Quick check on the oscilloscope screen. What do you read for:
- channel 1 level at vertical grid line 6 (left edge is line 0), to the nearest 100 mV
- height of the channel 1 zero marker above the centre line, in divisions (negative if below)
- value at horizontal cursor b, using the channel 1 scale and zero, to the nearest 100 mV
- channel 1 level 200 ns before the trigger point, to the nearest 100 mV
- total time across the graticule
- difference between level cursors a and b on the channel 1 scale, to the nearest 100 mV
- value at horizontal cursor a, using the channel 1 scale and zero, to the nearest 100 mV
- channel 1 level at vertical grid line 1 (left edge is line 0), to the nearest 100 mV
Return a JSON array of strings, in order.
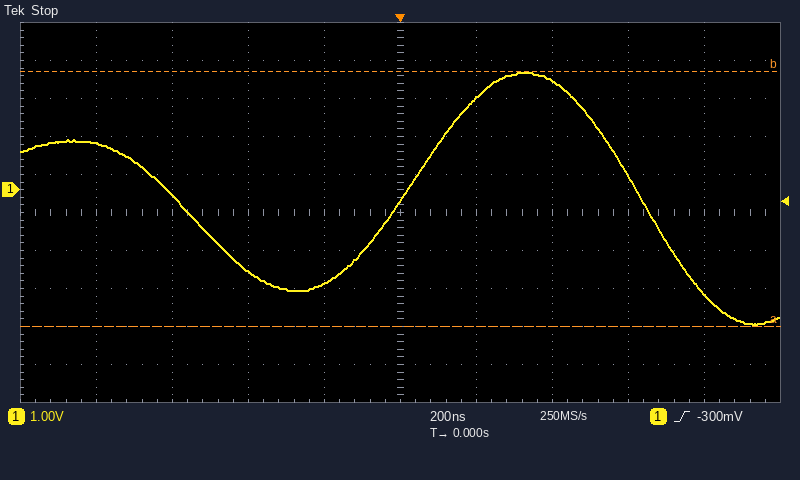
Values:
["2.4 V", "+0.6 div", "3.1 V", "-2.5 V", "2 µs", "6.7 V", "-3.6 V", "1.2 V"]
